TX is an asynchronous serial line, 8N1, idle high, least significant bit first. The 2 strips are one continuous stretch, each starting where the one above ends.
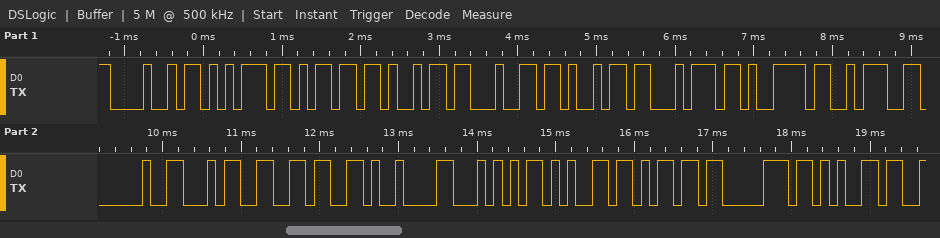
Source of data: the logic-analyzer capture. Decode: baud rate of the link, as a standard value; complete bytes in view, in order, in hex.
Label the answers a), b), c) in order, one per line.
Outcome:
a) 9600 baud
b) 48 75 6D 69 64 69 74 79 3A 20 34 36 09 54 65 6D 70 65
